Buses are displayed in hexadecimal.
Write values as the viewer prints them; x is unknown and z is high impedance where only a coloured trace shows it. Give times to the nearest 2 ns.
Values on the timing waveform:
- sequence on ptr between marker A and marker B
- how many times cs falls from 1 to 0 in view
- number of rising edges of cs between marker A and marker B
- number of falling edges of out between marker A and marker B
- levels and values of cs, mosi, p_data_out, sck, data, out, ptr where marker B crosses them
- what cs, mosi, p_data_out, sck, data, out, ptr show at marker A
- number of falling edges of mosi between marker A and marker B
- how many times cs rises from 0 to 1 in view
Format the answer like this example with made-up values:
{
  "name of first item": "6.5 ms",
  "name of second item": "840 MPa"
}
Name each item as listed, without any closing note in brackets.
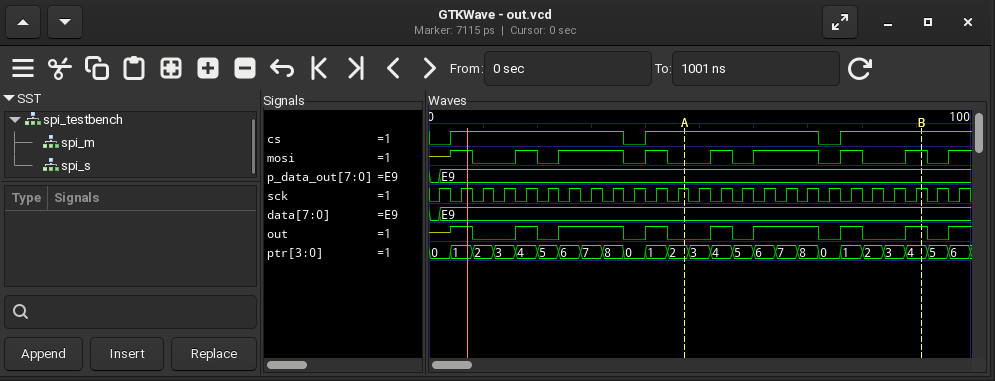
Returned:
{
  "sequence on ptr between marker A and marker B": "2, 3, 4, 5, 6, 7, 8, 0, 1, 2, 3, 4",
  "how many times cs falls from 1 to 0 in view": "2",
  "number of rising edges of cs between marker A and marker B": "1",
  "number of falling edges of out between marker A and marker B": "3",
  "levels and values of cs, mosi, p_data_out, sck, data, out, ptr where marker B crosses them": "cs=1, mosi=1, p_data_out=E9, sck=1, data=E9, out=1, ptr=4",
  "what cs, mosi, p_data_out, sck, data, out, ptr show at marker A": "cs=1, mosi=0, p_data_out=E9, sck=1, data=E9, out=0, ptr=2",
  "number of falling edges of mosi between marker A and marker B": "3",
  "how many times cs rises from 0 to 1 in view": "3"
}
